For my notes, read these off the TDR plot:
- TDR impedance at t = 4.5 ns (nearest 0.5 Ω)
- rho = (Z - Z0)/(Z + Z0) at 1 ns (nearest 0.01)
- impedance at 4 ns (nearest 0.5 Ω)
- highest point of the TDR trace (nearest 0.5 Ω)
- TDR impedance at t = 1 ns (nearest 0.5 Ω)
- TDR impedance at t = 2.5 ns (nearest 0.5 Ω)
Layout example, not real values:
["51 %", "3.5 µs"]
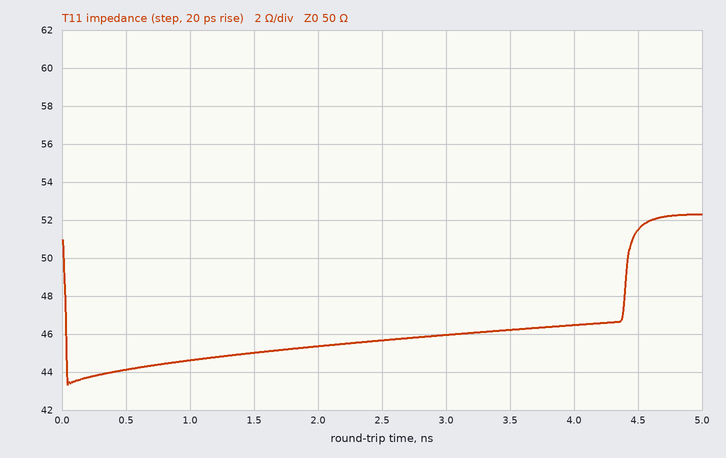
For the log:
["51.5 Ω", "-0.06", "46.5 Ω", "52.5 Ω", "44.5 Ω", "45.5 Ω"]
